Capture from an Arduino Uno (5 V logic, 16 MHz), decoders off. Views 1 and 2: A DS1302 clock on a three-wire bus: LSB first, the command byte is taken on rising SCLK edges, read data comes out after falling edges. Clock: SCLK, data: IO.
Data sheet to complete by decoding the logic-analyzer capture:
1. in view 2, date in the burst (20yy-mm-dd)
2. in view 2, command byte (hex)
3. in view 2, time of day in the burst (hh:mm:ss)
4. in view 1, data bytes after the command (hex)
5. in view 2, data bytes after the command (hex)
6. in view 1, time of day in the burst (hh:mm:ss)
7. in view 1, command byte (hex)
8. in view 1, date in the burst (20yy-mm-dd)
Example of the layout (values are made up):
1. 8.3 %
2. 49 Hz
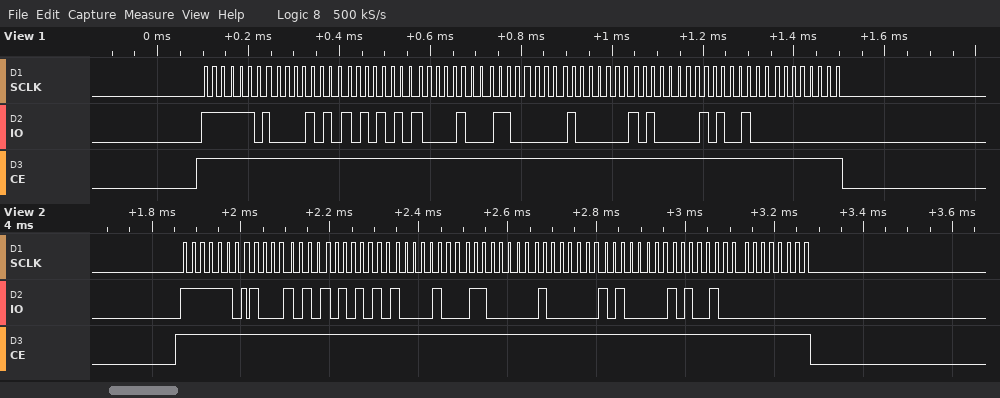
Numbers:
1. 2025-02-06
2. 0xBF
3. 21:55:51
4. 50 55 21 06 02 05 25 00
5. 51 55 21 06 02 05 25 00
6. 21:55:50
7. 0xBF
8. 2025-02-06
